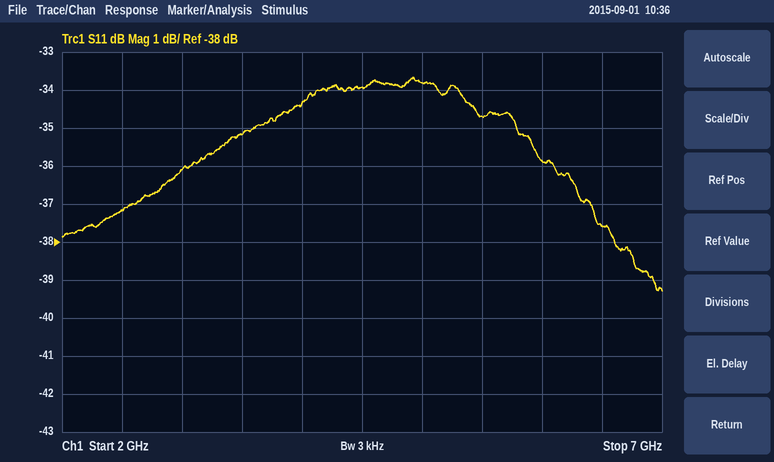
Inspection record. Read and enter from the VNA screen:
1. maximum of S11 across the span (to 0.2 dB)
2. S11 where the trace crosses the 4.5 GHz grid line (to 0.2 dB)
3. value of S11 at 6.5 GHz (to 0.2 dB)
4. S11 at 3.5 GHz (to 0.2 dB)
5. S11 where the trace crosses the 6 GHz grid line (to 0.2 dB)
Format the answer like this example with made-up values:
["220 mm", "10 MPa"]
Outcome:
["-33.6 dB", "-34.0 dB", "-37.6 dB", "-35.2 dB", "-35.8 dB"]
